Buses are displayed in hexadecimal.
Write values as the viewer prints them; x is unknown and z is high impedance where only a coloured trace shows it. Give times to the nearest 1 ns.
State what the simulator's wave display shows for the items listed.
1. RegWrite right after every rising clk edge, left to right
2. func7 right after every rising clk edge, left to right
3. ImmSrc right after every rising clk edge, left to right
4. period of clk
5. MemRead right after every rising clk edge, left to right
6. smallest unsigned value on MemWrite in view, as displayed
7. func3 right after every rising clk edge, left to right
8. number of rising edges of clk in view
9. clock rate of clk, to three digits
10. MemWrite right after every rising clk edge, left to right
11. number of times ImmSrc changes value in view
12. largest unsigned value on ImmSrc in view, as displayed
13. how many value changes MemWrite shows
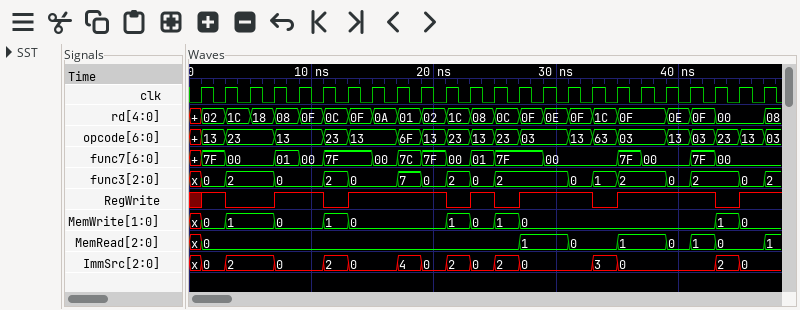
1 0 0 1 1 0 1 1 1 1 0 1 0 1 1 1 0 1 1 1 1 0 1 1
7F, 00, 00, 01, 00, 7F, 7F, 00, 7C, 7F, 00, 01, 7F, 7F, 00, 00, 00, 7F, 00, 00, 7F, 00, 00, 00
0, 2, 2, 0, 0, 2, 0, 0, 4, 0, 2, 0, 2, 0, 0, 0, 3, 0, 0, 0, 0, 2, 0, 0
2 ns
0, 0, 0, 0, 0, 0, 0, 0, 0, 0, 0, 0, 0, 1, 1, 0, 0, 1, 1, 0, 1, 0, 0, 1
0
0, 2, 2, 0, 0, 2, 0, 0, 7, 0, 2, 0, 2, 2, 2, 0, 1, 2, 2, 0, 2, 2, 0, 2
24
500 MHz
0, 1, 1, 0, 0, 1, 0, 0, 0, 0, 1, 0, 1, 0, 0, 0, 0, 0, 0, 0, 0, 1, 0, 0
15
4
11
